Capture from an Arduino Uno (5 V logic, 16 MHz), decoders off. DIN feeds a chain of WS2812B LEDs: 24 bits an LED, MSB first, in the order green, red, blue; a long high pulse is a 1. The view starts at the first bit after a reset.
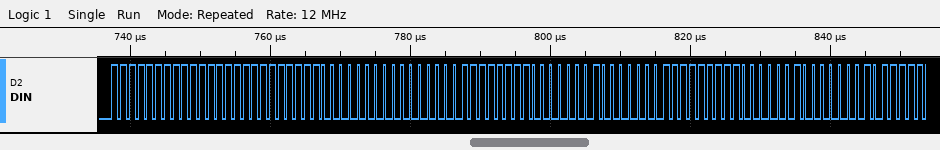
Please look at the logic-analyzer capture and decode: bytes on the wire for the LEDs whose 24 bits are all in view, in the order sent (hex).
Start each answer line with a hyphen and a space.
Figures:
- FF FF FF 00 00 FF 01 01 FF
